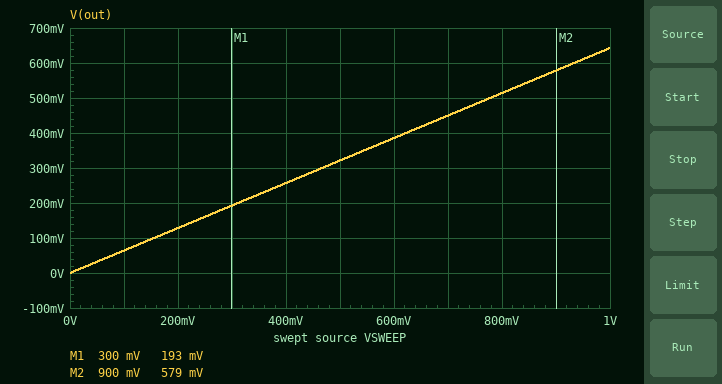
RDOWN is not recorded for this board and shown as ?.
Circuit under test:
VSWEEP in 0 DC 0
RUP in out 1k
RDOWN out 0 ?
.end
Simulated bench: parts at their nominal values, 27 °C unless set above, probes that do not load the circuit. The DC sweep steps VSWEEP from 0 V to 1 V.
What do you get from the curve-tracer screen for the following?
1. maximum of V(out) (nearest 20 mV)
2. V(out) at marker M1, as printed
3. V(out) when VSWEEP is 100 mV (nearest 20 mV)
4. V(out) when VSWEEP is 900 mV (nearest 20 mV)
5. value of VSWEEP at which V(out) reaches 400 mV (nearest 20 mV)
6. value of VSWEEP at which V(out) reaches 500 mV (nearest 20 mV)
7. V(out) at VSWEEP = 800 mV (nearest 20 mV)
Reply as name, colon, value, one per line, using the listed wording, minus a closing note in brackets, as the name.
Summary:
maximum of V(out): 640 mV
V(out) at marker M1, as printed: 193 mV
V(out) when VSWEEP is 100 mV: 60 mV
V(out) when VSWEEP is 900 mV: 580 mV
value of VSWEEP at which V(out) reaches 400 mV: 620 mV
value of VSWEEP at which V(out) reaches 500 mV: 780 mV
V(out) at VSWEEP = 800 mV: 520 mV
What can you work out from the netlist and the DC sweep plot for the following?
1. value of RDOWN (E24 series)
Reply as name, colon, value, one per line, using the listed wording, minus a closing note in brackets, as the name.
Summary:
value of RDOWN: 1.8 kΩ
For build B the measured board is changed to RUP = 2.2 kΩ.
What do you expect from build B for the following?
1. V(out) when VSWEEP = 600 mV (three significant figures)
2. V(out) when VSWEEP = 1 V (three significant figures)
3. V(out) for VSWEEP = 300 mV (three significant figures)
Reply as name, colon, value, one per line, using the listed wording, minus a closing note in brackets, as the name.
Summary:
V(out) when VSWEEP = 600 mV: 270 mV
V(out) when VSWEEP = 1 V: 450 mV
V(out) for VSWEEP = 300 mV: 135 mV
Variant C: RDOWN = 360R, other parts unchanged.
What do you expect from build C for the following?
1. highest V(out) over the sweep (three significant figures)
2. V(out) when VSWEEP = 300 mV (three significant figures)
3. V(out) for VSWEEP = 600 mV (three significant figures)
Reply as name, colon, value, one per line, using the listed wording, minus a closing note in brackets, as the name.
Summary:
highest V(out) over the sweep: 265 mV
V(out) when VSWEEP = 300 mV: 79.4 mV
V(out) for VSWEEP = 600 mV: 159 mV
